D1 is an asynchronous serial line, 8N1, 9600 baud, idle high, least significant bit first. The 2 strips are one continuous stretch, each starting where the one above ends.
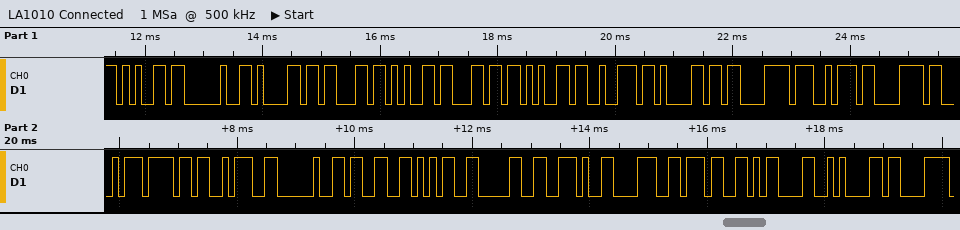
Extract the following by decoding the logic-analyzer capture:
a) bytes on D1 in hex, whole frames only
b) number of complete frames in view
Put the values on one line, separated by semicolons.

65 20 61 63 65 6C 65 72 61 C3 A7 C3 A3 6F 3A 20 33 35 30 2E 38 37 0D 0A C3; 25
